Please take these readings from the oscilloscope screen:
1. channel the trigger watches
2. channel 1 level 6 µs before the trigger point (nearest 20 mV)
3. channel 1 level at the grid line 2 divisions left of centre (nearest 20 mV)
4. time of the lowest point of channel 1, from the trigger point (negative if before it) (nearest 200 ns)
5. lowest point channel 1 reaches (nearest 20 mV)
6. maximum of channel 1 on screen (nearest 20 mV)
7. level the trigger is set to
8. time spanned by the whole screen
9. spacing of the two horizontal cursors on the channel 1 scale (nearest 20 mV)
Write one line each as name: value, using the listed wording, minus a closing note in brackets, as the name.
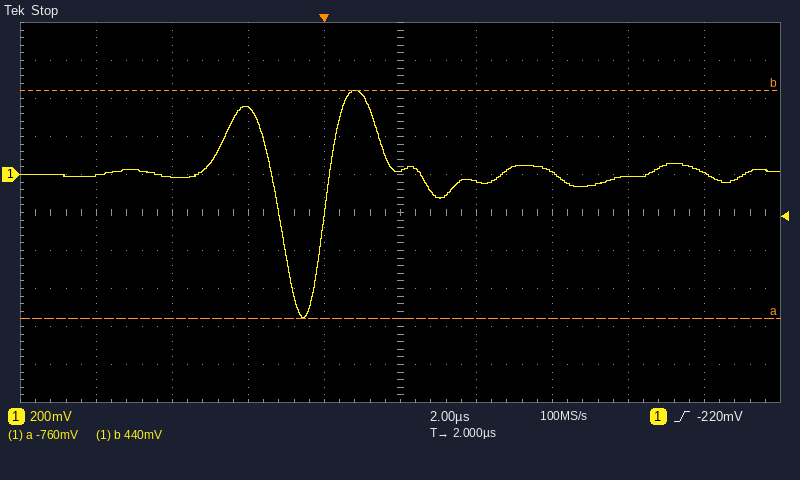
channel the trigger watches: channel 1
channel 1 level 6 µs before the trigger point: 0 mV
channel 1 level at the grid line 2 divisions left of centre: 340 mV
time of the lowest point of channel 1, from the trigger point (negative if before it): -600 ns
lowest point channel 1 reaches: -760 mV
maximum of channel 1 on screen: 440 mV
level the trigger is set to: -220 mV
time spanned by the whole screen: 20 µs
spacing of the two horizontal cursors on the channel 1 scale: 1.20 V
